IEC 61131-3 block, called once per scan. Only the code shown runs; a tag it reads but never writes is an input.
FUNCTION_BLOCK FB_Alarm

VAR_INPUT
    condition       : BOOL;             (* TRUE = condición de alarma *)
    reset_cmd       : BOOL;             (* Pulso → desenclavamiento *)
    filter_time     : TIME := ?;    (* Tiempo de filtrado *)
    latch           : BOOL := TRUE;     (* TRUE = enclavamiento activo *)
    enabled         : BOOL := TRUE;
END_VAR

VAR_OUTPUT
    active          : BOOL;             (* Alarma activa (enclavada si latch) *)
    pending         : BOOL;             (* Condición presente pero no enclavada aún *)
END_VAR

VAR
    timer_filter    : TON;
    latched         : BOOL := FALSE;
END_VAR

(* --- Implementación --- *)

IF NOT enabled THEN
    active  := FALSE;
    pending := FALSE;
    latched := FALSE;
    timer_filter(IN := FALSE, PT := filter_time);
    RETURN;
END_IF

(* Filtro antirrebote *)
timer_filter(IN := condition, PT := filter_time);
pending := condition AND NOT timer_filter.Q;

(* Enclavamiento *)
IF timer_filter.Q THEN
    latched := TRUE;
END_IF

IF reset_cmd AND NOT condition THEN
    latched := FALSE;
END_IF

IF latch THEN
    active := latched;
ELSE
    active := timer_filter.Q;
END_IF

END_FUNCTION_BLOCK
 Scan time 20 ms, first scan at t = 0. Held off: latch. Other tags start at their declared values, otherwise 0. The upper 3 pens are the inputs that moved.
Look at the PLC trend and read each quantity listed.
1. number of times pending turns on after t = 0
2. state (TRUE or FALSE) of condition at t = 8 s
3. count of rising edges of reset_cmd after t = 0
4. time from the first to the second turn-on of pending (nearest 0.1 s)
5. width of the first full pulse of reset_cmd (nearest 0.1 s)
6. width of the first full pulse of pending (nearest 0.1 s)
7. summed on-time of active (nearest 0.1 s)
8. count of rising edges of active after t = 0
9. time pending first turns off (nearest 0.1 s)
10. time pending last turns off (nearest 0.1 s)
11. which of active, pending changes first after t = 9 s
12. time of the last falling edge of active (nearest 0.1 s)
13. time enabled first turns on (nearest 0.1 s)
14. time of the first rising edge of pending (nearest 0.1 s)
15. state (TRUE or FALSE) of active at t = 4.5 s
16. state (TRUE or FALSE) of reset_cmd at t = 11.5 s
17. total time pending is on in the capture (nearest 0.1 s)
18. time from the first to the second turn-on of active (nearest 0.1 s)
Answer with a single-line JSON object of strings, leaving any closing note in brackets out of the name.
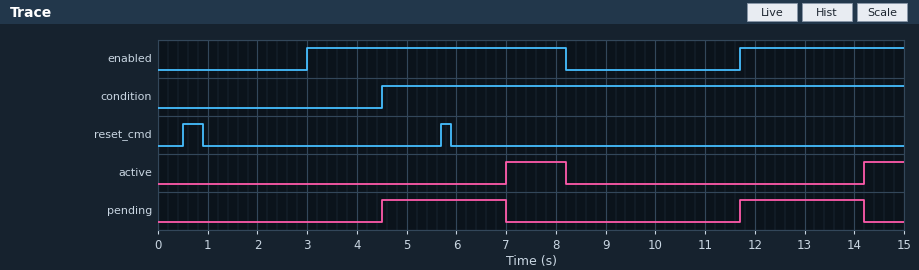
{"number of times pending turns on after t = 0": "2", "state (TRUE or FALSE) of condition at t = 8 s": "TRUE", "count of rising edges of reset_cmd after t = 0": "2", "time from the first to the second turn-on of pending": "7.2 s", "width of the first full pulse of reset_cmd": "0.4 s", "width of the first full pulse of pending": "2.5 s", "summed on-time of active": "2.0 s", "count of rising edges of active after t = 0": "2", "time pending first turns off": "7.0 s", "time pending last turns off": "14.2 s", "which of active, pending changes first after t = 9 s": "pending", "time of the last falling edge of active": "8.2 s", "time enabled first turns on": "3.0 s", "time of the first rising edge of pending": "4.5 s", "state (TRUE or FALSE) of active at t = 4.5 s": "FALSE", "state (TRUE or FALSE) of reset_cmd at t = 11.5 s": "FALSE", "total time pending is on in the capture": "5.0 s", "time from the first to the second turn-on of active": "7.2 s"}
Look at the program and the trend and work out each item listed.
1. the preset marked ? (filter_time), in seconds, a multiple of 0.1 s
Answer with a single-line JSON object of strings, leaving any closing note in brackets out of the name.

{"the preset marked ? (filter_time), in seconds, a multiple of 0.1 s": "2.5 s"}
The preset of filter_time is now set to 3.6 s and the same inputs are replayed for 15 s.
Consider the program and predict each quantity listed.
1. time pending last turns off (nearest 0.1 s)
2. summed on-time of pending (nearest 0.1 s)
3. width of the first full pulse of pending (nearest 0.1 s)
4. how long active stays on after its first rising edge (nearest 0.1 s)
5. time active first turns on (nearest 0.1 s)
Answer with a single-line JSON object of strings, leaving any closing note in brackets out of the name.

{"time pending last turns off": "8.1 s", "summed on-time of pending": "6.9 s", "width of the first full pulse of pending": "3.6 s", "how long active stays on after its first rising edge": "0.1 s", "time active first turns on": "8.1 s"}
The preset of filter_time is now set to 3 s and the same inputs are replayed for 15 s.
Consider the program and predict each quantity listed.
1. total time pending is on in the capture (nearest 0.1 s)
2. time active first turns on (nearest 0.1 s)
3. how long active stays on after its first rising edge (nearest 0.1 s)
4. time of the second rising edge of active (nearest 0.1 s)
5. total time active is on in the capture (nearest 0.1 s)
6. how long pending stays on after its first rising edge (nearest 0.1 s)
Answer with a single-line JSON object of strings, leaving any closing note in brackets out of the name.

{"total time pending is on in the capture": "6.0 s", "time active first turns on": "7.5 s", "how long active stays on after its first rising edge": "0.7 s", "time of the second rising edge of active": "14.7 s", "total time active is on in the capture": "1.0 s", "how long pending stays on after its first rising edge": "3.0 s"}
